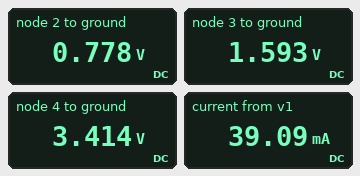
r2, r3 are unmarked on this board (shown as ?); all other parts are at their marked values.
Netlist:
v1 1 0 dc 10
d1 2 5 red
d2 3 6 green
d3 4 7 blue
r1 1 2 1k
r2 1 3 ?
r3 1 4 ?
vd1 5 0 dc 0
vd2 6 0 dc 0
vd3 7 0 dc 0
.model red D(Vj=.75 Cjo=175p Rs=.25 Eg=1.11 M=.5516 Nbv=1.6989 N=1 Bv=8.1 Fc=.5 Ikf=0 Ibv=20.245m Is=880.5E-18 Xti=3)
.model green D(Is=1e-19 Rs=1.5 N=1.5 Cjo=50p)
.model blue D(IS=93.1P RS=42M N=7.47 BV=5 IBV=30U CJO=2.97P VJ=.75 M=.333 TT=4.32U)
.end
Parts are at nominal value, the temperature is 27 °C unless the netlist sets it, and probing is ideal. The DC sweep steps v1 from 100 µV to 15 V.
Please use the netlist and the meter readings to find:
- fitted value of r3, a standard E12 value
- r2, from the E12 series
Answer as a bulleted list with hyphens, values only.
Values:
- 1.5 kΩ
- 330 Ω
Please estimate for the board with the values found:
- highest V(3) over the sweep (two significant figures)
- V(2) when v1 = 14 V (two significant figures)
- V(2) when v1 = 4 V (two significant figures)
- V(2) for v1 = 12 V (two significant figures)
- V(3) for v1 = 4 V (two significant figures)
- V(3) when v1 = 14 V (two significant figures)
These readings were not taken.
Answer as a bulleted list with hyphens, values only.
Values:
- 1.6 V
- 790 mV
- 750 mV
- 780 mV
- 1.5 V
- 1.6 V
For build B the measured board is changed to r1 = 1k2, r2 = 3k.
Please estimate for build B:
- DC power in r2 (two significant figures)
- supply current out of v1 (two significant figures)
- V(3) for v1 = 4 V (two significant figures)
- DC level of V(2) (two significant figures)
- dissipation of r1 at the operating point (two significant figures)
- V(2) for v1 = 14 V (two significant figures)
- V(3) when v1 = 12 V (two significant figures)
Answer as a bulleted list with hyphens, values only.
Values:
- 24 mW
- 15 mA
- 1.4 V
- 770 mV
- 71 mW
- 780 mV
- 1.5 V
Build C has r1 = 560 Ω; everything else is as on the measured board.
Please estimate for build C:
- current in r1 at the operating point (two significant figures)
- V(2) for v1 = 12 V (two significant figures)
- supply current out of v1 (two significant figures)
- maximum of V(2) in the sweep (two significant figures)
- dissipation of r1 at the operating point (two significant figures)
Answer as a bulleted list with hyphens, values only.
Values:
- 16 mA
- 800 mV
- 46 mA
- 810 mV
- 150 mW
